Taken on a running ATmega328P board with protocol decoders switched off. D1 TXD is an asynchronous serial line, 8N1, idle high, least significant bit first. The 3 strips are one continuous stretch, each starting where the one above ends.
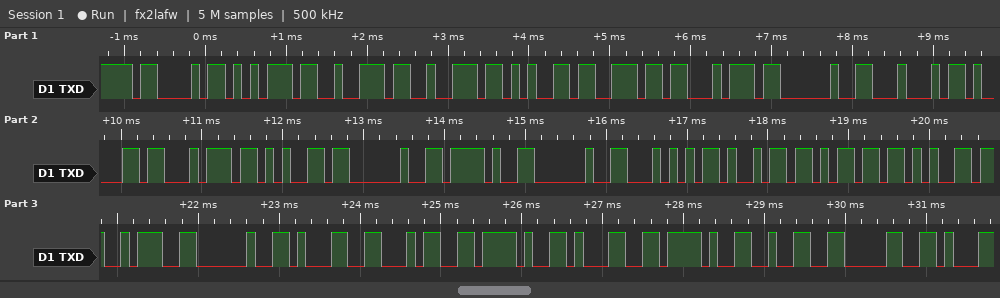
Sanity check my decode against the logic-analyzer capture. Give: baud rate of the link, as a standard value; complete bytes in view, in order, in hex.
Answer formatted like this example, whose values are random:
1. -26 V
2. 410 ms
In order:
1. 9600 baud
2. 43 75 72 72 65 6E 74 20 44 61 74 65 20 2F 20 54 69 6D 65 3A 20 31 34 2F 31 2F 32 30
